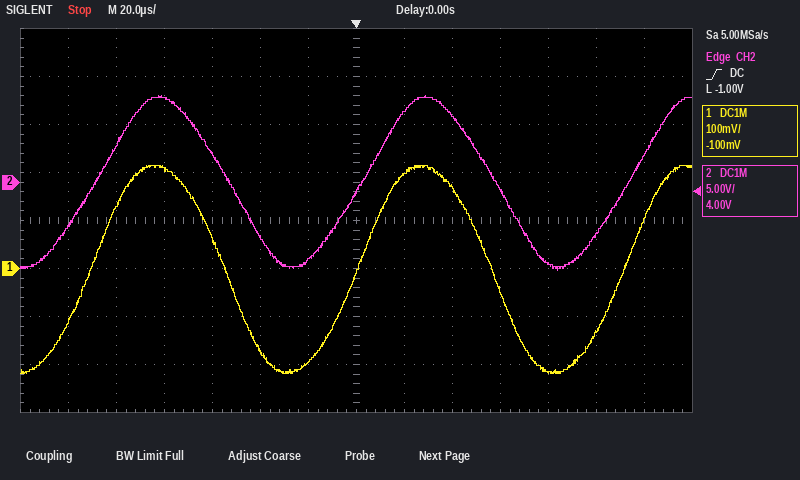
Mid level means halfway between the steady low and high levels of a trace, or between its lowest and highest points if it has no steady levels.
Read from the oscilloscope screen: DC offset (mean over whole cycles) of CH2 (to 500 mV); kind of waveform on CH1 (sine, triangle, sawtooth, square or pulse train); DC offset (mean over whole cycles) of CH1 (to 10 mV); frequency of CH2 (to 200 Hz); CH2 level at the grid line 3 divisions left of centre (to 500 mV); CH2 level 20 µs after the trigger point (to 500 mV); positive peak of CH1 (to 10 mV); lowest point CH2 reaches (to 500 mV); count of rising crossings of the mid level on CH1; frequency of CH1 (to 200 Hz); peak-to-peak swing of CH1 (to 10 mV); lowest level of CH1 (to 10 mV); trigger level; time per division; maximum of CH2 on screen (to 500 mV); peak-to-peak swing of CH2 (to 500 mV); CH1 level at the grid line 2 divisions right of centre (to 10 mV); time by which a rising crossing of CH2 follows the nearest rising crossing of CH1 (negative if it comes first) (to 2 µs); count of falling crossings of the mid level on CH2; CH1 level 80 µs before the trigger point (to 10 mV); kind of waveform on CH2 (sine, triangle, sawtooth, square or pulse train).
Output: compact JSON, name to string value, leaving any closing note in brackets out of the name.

{"DC offset (mean over whole cycles) of CH2": "0.0 V", "kind of waveform on CH1": "sine", "DC offset (mean over whole cycles) of CH1": "0 mV", "frequency of CH2": "9.0 kHz", "CH2 level at the grid line 3 divisions left of centre": "3.0 V", "CH2 level 20 µs after the trigger point": "7.5 V", "positive peak of CH1": "210 mV", "lowest point CH2 reaches": "-9.0 V", "count of rising crossings of the mid level on CH1": "3", "frequency of CH1": "9.0 kHz", "peak-to-peak swing of CH1": "430 mV", "lowest level of CH1": "-220 mV", "trigger level": "-1.00 V", "time per division": "20 µs", "maximum of CH2 on screen": "9.0 V", "peak-to-peak swing of CH2": "18.0 V", "CH1 level at the grid line 2 divisions right of centre": "170 mV", "time by which a rising crossing of CH2 follows the nearest rising crossing of CH1 (negative if it comes first)": "+2 µs", "count of falling crossings of the mid level on CH2": "2", "CH1 level 80 µs before the trigger point": "210 mV", "kind of waveform on CH2": "sine"}
